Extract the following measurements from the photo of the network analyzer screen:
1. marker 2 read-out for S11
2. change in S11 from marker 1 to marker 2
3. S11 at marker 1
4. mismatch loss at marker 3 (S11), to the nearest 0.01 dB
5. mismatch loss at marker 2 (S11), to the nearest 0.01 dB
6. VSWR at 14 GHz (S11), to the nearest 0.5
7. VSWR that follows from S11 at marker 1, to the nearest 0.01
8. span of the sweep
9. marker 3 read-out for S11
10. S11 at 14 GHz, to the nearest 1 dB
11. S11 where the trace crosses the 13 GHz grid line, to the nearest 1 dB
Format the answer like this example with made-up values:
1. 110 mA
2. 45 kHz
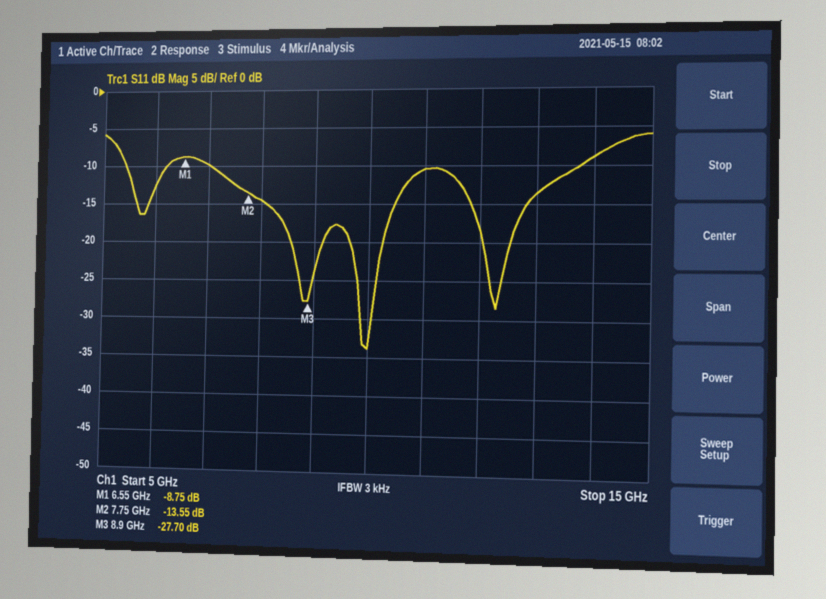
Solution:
1. -13.55 dB
2. -4.80 dB
3. -8.75 dB
4. 0.01 dB
5. 0.20 dB
6. 2.0
7. 2.15
8. 10 GHz
9. -27.70 dB
10. -9 dB
11. -14 dB
